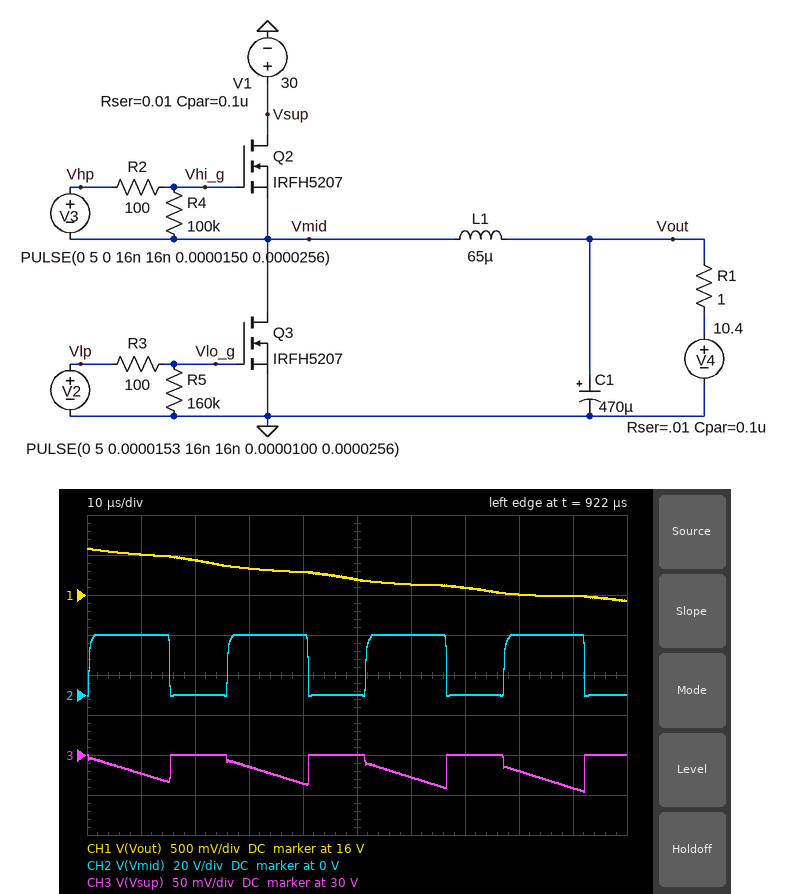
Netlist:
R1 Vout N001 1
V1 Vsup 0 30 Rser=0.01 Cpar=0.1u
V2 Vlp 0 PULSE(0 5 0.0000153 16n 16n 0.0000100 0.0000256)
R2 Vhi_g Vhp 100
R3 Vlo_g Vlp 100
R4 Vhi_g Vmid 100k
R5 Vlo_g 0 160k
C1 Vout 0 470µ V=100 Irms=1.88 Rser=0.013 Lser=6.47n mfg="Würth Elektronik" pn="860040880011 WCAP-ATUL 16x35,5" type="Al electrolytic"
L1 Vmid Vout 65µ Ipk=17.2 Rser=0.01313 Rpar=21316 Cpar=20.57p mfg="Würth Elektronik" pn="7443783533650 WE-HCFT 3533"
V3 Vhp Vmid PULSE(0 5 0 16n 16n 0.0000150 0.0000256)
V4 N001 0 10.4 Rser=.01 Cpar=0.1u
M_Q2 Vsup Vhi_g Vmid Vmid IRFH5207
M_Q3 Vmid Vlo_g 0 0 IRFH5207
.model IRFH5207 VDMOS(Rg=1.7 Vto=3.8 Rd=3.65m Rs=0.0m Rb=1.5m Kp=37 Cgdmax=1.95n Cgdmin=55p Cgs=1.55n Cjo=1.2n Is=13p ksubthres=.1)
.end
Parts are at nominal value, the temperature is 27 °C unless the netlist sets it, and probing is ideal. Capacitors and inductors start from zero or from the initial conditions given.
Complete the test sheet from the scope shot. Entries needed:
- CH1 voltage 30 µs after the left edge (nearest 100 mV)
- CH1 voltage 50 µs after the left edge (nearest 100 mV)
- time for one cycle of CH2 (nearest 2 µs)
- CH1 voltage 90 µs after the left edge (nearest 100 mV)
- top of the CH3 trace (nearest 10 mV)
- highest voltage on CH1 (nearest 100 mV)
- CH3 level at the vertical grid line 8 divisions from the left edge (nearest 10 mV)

16.3 V
16.2 V
26 µs
16.0 V
30.00 V
16.6 V
29.98 V
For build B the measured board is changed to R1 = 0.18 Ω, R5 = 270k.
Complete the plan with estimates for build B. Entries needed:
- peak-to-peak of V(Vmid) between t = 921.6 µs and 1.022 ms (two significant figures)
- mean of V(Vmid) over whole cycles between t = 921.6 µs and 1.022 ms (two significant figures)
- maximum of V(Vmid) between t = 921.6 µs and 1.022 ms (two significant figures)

30 V
15 V
29 V
